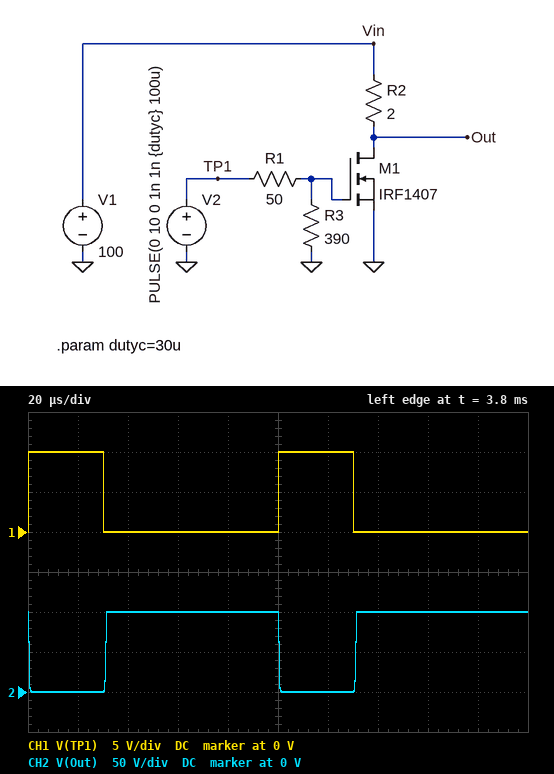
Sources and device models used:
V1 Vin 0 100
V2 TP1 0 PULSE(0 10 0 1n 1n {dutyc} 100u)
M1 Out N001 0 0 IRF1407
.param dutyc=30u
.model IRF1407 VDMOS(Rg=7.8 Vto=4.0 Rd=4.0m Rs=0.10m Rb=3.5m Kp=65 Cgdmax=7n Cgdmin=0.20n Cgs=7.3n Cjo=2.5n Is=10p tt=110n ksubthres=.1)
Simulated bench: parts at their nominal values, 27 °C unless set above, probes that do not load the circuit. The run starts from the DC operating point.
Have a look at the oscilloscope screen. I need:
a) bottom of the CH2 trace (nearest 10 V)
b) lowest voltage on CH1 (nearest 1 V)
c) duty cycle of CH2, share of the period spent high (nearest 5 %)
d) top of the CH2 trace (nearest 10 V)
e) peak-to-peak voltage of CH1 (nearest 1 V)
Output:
0 V
0 V
70 %
100 V
10 V
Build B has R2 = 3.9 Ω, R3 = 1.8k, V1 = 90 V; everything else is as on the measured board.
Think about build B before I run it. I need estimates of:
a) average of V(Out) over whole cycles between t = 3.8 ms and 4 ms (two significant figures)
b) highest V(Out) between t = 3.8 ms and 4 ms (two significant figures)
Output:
62 V
90 V
